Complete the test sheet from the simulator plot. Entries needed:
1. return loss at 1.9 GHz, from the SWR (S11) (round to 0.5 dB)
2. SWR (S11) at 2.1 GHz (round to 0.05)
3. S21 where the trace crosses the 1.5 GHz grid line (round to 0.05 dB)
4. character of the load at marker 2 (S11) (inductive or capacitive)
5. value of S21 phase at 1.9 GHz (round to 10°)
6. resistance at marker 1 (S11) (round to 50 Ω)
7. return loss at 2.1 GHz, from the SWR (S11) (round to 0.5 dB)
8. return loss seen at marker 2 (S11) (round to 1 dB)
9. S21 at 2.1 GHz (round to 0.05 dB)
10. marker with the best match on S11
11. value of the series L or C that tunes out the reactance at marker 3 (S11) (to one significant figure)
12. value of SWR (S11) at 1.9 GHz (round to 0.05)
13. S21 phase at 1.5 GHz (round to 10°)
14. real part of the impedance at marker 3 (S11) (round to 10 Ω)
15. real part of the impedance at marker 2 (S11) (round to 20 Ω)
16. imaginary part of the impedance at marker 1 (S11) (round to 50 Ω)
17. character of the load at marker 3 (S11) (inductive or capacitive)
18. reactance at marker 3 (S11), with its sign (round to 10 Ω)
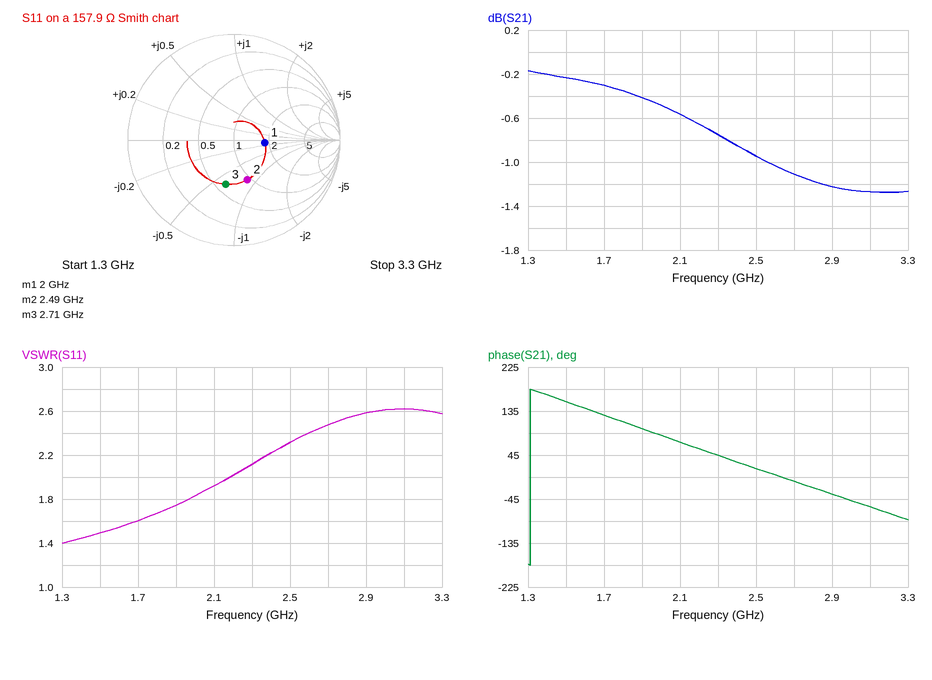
11.5 dB
1.90
-0.25 dB
capacitive
100°
300 Ω
10.0 dB
8 dB
-0.55 dB
marker 1
6 nH
1.75
150°
100 Ω
140 Ω
0 Ω
capacitive
-100 Ω
